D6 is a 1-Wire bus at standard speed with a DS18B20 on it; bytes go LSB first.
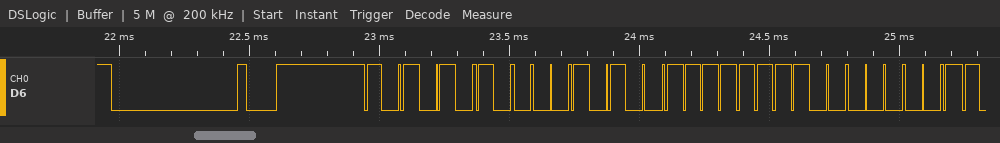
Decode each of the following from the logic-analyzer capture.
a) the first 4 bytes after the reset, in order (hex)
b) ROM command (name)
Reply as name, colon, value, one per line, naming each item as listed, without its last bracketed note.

the first 4 bytes after the reset, in order: 55 28 FF 80
ROM command: Match ROM
